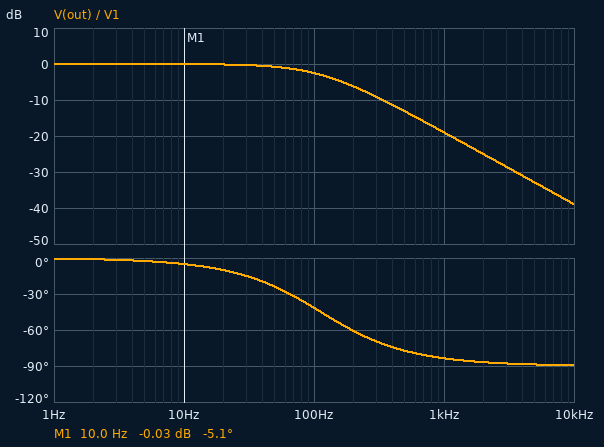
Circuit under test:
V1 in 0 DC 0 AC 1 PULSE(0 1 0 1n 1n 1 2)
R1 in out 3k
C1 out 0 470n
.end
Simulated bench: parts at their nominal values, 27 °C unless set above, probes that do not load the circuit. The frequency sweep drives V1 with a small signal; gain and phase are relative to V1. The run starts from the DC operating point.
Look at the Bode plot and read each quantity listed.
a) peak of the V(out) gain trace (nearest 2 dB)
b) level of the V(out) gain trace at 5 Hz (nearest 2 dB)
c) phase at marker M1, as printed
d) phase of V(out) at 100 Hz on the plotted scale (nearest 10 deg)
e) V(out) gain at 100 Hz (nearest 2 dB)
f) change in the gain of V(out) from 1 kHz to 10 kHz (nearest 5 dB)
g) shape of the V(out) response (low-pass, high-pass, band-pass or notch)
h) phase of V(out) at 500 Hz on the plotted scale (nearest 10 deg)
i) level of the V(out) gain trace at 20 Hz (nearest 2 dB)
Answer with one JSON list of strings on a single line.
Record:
["0 dB", "0 dB", "-5.1 deg", "-40 deg", "-2 dB", "-20 dB", "low-pass", "-80 deg", "0 dB"]
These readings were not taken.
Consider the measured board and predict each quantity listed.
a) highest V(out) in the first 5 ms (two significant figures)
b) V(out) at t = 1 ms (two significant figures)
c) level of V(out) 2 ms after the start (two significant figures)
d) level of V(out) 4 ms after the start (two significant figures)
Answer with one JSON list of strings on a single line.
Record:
["970 mV", "510 mV", "760 mV", "940 mV"]
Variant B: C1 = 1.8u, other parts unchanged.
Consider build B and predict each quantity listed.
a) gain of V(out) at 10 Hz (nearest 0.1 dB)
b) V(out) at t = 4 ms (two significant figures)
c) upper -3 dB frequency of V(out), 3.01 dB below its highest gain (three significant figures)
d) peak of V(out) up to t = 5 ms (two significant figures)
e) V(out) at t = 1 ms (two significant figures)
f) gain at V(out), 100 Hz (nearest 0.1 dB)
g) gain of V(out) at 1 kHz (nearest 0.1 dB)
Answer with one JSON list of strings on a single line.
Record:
["-0.5 dB", "520 mV", "29.5 Hz", "600 mV", "170 mV", "-11.0 dB", "-30.6 dB"]
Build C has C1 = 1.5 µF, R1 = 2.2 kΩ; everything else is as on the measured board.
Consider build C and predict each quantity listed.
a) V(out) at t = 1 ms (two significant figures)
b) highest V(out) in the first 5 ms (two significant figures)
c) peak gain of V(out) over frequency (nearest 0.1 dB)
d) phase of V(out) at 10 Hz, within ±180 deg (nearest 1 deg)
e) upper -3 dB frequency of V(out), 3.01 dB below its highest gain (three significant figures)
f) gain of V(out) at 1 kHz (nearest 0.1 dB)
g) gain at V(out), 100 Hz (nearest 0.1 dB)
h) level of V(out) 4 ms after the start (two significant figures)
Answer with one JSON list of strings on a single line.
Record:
["260 mV", "780 mV", "0 dB", "-12 deg", "48.2 Hz", "-26.3 dB", "-7.2 dB", "700 mV"]
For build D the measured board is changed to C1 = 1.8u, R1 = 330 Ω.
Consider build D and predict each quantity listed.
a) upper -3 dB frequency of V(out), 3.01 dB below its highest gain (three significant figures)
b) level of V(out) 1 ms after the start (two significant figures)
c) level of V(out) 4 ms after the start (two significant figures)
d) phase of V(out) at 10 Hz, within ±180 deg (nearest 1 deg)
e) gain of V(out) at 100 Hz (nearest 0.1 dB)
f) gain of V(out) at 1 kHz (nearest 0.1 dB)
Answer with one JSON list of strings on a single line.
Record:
["268 Hz", "810 mV", "1.0 V", "-2 deg", "-0.6 dB", "-11.7 dB"]
